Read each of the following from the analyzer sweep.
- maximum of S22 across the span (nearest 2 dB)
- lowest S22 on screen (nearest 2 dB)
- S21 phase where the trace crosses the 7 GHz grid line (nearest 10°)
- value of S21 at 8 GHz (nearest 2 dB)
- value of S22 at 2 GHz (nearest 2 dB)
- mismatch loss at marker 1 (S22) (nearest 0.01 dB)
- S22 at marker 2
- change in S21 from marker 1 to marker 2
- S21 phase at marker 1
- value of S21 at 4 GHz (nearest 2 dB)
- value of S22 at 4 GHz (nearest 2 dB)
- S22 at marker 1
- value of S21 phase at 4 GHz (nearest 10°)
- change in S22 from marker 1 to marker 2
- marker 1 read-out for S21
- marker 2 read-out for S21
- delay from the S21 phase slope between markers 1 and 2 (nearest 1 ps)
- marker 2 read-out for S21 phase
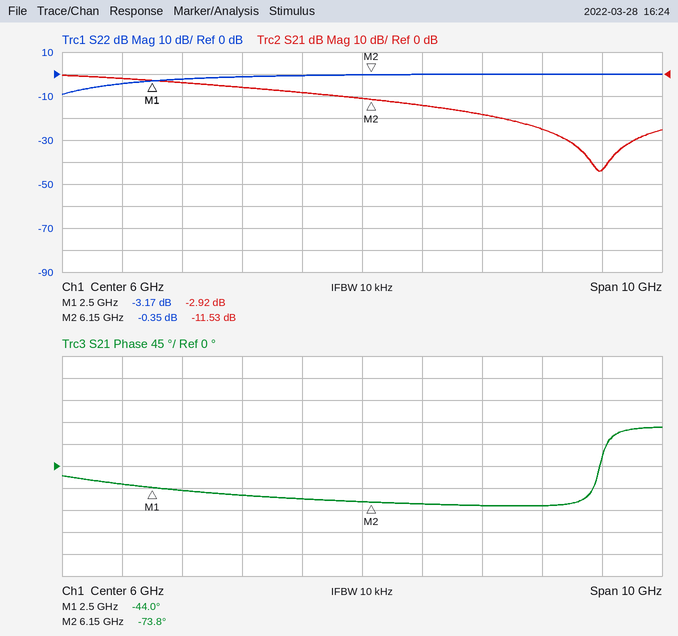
0 dB
-10 dB
-80°
-18 dB
-4 dB
2.86 dB
-0.35 dB
-8.61 dB
-44.0°
-6 dB
-2 dB
-3.17 dB
-60°
2.82 dB
-2.92 dB
-11.53 dB
23 ps
-73.8°
